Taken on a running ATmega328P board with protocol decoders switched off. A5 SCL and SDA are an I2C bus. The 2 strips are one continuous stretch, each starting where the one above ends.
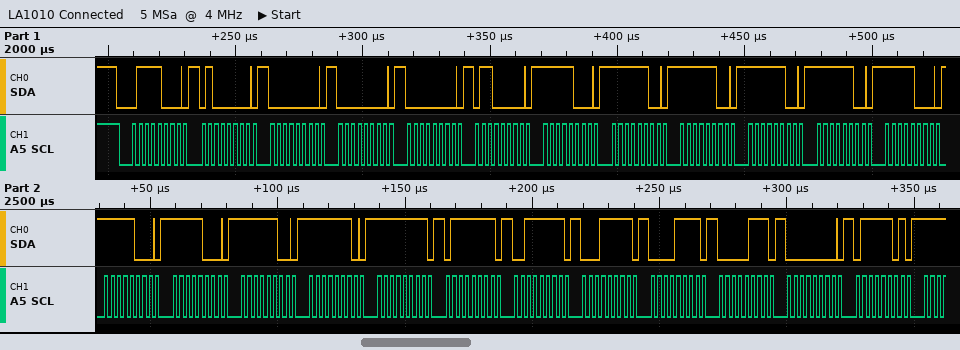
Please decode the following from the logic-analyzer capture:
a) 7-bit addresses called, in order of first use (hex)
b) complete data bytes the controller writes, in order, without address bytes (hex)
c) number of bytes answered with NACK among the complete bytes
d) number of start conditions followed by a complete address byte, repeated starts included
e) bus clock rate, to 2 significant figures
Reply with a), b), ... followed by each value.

a) 0x3C
b) 40 00 00 00 60 F8 FC FC FC FC F8 F8 F8 FC FE FF 7F 3F 1F 0F 07 00 7D
c) 0
d) 1
e) 400 kHz
